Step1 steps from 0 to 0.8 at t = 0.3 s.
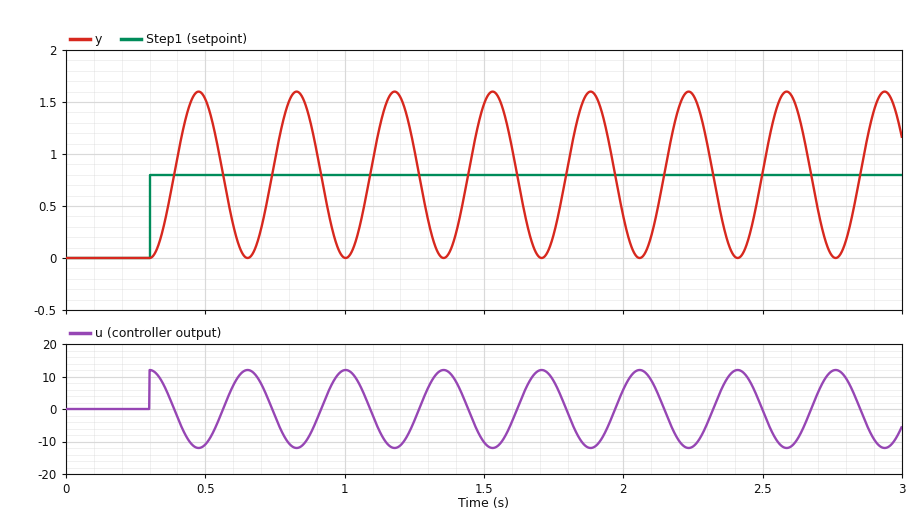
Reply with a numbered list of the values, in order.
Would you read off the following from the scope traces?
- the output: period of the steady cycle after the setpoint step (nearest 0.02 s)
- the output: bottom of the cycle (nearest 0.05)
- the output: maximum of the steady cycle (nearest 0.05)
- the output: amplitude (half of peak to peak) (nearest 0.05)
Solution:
1. 0.36 s
2. 0.00
3. 1.60
4. 0.80
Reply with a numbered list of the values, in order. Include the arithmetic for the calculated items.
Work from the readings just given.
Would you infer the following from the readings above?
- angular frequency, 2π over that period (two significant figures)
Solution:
1. 2π / 0.36 = 17 rad/s
